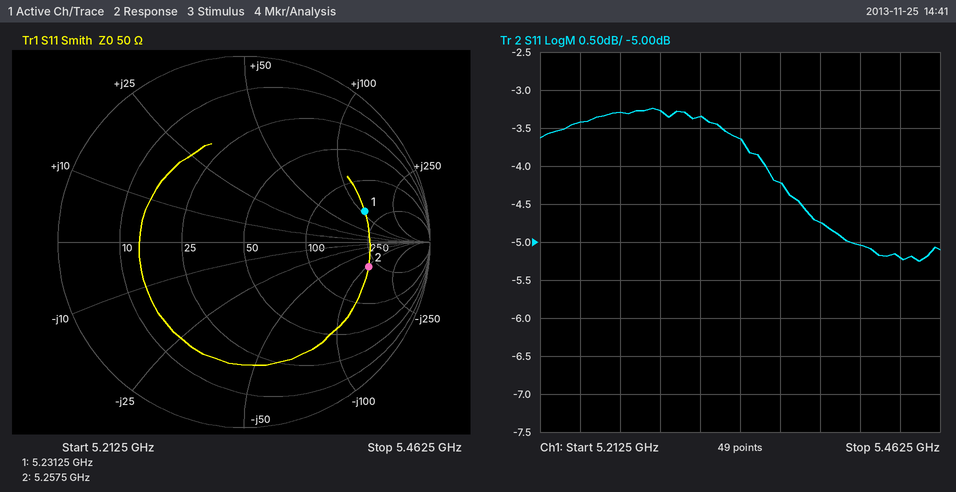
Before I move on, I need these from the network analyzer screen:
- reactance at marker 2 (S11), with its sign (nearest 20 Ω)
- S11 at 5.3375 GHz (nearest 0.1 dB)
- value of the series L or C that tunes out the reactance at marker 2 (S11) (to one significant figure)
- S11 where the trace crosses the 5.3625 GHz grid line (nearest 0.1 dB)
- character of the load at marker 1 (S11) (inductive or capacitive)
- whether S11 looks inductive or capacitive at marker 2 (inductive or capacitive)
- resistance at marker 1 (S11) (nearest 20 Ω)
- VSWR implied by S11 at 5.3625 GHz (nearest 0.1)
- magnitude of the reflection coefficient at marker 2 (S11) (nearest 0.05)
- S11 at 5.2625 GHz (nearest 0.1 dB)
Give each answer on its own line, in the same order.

-100 Ω
-3.6 dB
3 nH
-4.2 dB
inductive
capacitive
180 Ω
4.2
0.70
-3.3 dB
